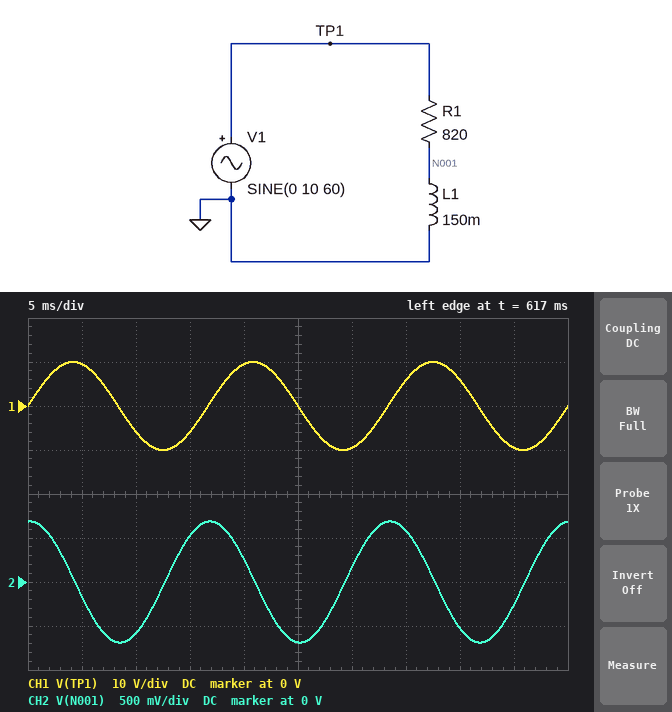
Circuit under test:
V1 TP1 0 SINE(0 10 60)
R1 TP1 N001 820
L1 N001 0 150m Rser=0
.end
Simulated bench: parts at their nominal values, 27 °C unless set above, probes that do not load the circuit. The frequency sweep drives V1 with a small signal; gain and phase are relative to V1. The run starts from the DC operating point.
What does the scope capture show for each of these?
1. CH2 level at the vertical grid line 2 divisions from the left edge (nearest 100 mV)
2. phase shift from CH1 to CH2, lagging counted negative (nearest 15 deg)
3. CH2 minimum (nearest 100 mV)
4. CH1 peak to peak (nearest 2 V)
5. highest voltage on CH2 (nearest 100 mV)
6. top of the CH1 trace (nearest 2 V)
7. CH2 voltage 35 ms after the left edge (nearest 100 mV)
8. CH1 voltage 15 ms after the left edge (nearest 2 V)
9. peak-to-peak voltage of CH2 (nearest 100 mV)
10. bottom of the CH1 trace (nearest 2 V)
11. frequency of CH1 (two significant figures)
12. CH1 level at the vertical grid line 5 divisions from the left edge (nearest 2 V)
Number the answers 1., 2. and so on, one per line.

1. -600 mV
2. 90 deg
3. -700 mV
4. 20 V
5. 700 mV
6. 10 V
7. 600 mV
8. -6 V
9. 1.4 V
10. -10 V
11. 60 Hz
12. 0 V
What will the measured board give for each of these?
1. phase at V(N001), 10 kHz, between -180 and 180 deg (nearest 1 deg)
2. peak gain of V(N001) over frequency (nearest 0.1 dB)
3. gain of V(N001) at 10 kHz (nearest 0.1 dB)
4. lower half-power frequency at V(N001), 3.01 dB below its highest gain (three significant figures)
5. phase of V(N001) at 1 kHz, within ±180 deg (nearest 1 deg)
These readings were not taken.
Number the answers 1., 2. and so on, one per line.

1. 5 deg
2. 0 dB
3. 0 dB
4. 870 Hz
5. 41 deg
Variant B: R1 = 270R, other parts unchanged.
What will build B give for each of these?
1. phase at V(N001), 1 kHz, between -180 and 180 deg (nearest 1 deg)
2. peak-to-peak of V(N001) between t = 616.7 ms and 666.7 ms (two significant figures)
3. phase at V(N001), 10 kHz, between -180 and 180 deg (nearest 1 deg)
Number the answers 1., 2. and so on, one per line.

1. 16 deg
2. 4.1 V
3. 2 deg
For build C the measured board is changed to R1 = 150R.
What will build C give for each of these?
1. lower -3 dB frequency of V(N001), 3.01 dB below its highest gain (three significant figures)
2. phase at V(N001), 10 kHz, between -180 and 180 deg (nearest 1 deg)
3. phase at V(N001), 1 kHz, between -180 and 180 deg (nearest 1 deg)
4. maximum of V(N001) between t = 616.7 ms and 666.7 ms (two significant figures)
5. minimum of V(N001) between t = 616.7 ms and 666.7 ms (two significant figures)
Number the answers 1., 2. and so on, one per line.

1. 159 Hz
2. 1 deg
3. 9 deg
4. 3.5 V
5. -3.5 V
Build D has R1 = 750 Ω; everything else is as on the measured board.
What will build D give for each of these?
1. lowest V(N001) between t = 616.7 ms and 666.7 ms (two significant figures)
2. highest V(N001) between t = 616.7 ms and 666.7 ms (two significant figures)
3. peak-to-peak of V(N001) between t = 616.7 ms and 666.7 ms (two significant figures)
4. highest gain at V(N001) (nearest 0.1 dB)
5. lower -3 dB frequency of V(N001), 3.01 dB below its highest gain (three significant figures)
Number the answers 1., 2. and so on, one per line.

1. -750 mV
2. 750 mV
3. 1.5 V
4. 0 dB
5. 796 Hz
